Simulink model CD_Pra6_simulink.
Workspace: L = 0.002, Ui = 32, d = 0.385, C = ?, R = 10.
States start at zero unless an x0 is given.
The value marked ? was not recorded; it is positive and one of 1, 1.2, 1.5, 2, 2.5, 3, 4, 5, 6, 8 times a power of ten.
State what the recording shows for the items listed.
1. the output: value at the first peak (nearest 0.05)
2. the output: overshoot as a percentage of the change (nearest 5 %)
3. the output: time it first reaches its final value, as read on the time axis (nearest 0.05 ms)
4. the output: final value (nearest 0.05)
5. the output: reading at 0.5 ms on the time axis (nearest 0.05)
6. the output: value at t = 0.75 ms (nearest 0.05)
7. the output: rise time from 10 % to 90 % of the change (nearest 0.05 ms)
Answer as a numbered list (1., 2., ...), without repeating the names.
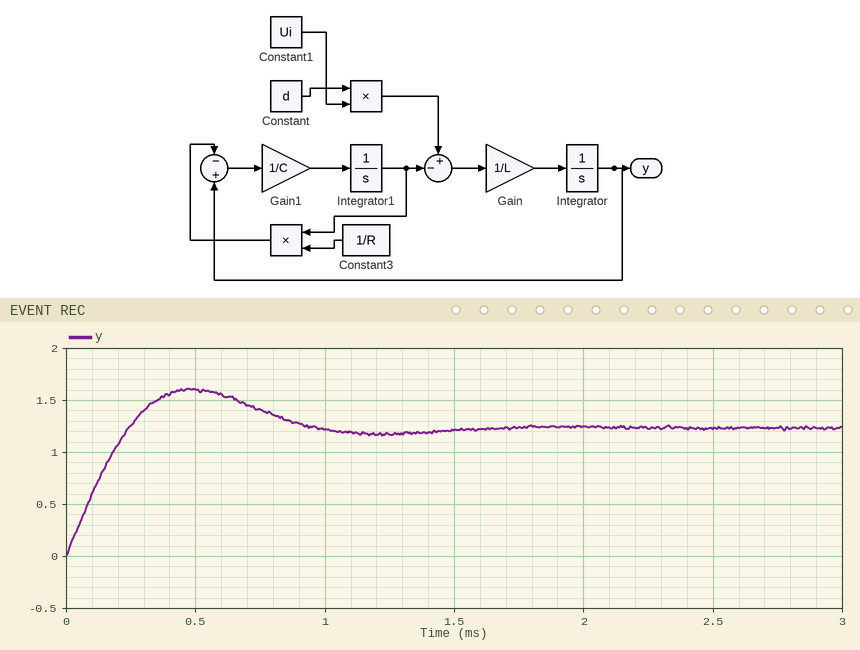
1. 1.60
2. 30 %
3. 0.25 ms
4. 1.25
5. 1.60
6. 1.40
7. 0.20 ms
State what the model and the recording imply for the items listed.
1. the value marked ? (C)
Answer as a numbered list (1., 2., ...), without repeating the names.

1. 2e-05
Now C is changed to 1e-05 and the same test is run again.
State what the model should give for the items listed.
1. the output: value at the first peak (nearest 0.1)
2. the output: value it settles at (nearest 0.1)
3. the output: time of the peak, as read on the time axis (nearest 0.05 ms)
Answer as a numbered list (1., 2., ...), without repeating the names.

1. 1.3
2. 1.2
3. 0.45 ms
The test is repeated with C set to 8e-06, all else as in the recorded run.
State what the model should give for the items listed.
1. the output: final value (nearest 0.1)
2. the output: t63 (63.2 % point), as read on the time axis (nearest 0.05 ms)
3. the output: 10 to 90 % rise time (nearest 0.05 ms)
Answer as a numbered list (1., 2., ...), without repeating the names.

1. 1.2
2. 0.15 ms
3. 0.25 ms
